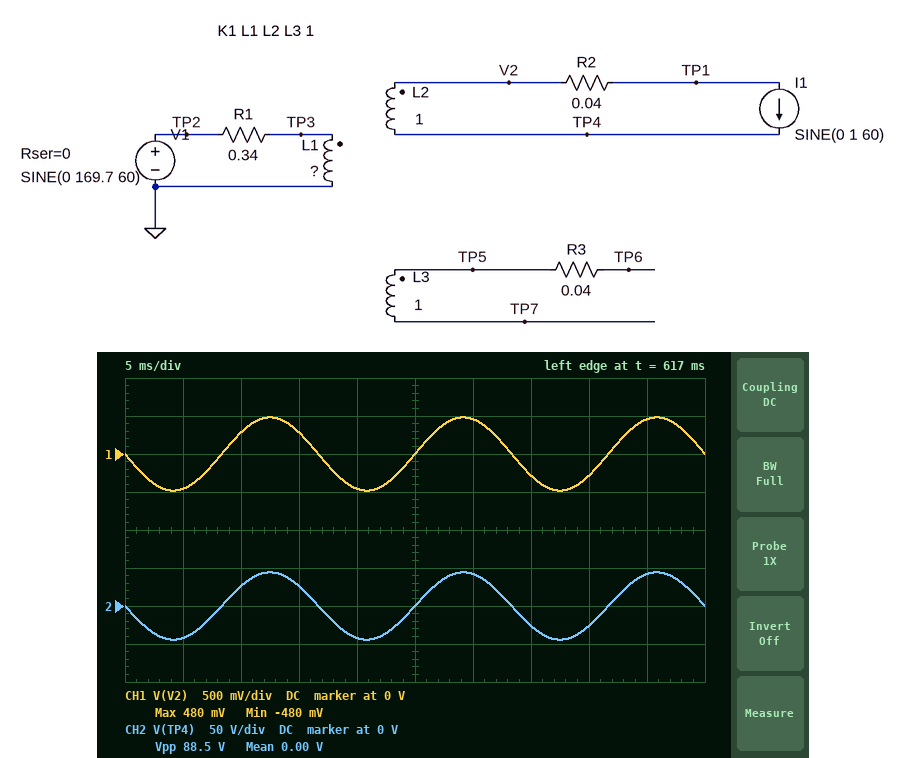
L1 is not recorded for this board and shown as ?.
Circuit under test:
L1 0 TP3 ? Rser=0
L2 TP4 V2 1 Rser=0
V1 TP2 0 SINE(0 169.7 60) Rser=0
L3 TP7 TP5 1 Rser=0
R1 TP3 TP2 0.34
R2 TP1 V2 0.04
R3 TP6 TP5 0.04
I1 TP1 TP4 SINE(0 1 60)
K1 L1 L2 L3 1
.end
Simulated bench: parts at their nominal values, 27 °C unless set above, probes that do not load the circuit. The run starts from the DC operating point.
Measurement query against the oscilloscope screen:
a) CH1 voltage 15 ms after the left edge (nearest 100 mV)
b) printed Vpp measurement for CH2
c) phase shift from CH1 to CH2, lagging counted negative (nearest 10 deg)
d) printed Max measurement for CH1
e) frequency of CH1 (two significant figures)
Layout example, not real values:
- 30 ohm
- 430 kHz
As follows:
- 300 mV
- 88.5 V
- 0 deg
- 480 mV
- 60 Hz
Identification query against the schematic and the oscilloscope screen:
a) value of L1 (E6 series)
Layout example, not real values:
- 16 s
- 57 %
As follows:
- 15 H
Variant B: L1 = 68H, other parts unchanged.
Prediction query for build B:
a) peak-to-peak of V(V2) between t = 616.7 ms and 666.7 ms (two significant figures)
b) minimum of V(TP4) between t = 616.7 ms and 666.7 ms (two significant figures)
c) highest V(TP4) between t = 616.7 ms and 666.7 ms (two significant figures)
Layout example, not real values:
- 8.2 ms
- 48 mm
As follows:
- 960 mV
- -21 V
- 21 V
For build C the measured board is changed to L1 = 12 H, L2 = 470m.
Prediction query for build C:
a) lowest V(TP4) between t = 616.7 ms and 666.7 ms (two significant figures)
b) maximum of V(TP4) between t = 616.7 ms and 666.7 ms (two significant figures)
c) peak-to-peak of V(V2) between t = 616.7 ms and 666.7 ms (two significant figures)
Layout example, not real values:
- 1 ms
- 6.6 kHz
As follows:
- -34 V
- 34 V
- 960 mV
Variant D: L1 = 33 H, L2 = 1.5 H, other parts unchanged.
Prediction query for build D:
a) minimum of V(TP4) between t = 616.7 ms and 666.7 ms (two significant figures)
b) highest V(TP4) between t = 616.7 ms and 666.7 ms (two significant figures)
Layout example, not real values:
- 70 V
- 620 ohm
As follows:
- -37 V
- 37 V
